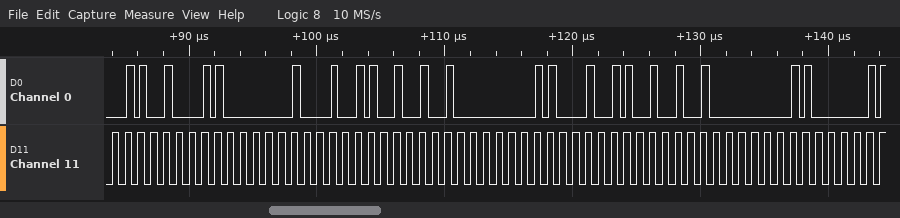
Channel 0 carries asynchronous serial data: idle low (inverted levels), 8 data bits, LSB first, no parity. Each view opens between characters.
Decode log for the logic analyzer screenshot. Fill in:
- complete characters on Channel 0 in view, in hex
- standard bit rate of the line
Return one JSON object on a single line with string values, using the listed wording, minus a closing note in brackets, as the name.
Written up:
{"complete characters on Channel 0 in view, in hex": "DD, FD, DF, DD, F7, 7D, DD, F7, FD", "standard bit rate of the line": "2000000 baud"}
